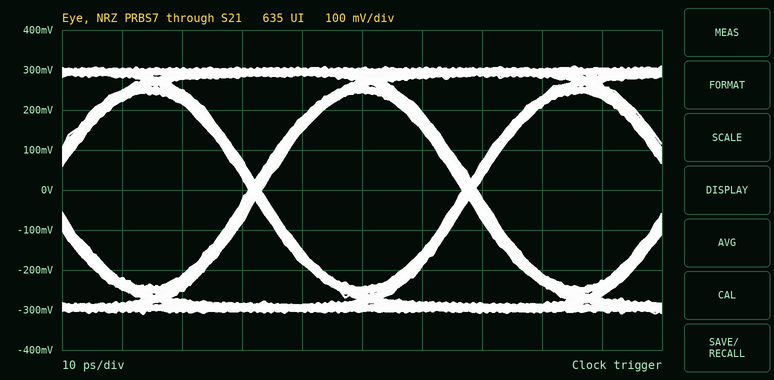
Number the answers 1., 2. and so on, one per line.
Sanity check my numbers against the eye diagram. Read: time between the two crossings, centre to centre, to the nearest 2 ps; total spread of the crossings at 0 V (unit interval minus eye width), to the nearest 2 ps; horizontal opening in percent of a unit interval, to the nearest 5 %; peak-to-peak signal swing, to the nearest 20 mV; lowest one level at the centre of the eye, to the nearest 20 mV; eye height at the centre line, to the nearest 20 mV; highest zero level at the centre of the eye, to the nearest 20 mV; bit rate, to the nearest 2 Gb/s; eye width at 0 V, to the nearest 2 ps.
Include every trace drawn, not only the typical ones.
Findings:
1. 36 ps
2. 2 ps
3. 95 %
4. 620 mV
5. 240 mV
6. 480 mV
7. -240 mV
8. 28 Gb/s
9. 34 ps
